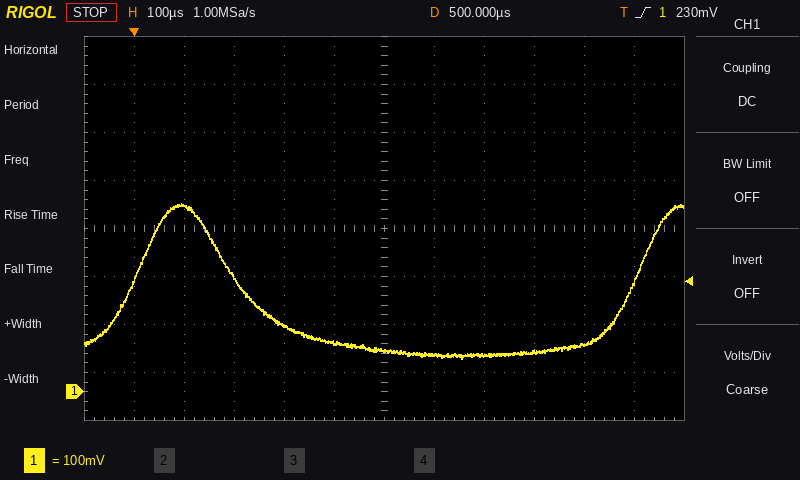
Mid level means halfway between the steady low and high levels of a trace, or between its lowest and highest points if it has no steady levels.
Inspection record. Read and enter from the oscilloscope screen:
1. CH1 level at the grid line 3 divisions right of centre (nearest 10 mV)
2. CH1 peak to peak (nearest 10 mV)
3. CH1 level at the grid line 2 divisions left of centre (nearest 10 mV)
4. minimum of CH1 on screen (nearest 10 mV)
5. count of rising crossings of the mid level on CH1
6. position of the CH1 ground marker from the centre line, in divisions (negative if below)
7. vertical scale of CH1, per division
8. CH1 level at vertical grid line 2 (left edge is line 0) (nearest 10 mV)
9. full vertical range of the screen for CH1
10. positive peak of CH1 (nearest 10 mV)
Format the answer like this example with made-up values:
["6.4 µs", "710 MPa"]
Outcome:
["80 mV", "320 mV", "140 mV", "70 mV", "2", "-3.4 div", "100 mV", "390 mV", "800 mV", "390 mV"]
